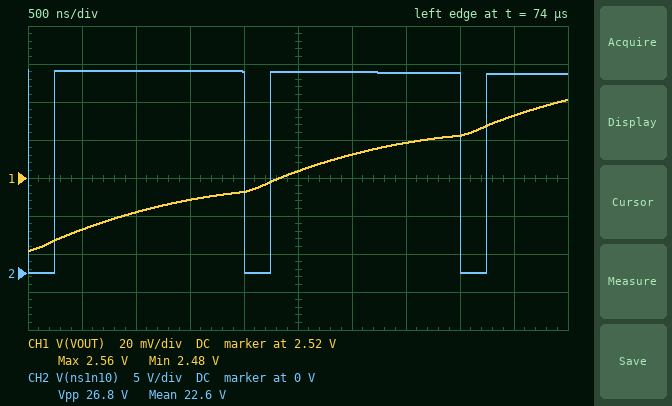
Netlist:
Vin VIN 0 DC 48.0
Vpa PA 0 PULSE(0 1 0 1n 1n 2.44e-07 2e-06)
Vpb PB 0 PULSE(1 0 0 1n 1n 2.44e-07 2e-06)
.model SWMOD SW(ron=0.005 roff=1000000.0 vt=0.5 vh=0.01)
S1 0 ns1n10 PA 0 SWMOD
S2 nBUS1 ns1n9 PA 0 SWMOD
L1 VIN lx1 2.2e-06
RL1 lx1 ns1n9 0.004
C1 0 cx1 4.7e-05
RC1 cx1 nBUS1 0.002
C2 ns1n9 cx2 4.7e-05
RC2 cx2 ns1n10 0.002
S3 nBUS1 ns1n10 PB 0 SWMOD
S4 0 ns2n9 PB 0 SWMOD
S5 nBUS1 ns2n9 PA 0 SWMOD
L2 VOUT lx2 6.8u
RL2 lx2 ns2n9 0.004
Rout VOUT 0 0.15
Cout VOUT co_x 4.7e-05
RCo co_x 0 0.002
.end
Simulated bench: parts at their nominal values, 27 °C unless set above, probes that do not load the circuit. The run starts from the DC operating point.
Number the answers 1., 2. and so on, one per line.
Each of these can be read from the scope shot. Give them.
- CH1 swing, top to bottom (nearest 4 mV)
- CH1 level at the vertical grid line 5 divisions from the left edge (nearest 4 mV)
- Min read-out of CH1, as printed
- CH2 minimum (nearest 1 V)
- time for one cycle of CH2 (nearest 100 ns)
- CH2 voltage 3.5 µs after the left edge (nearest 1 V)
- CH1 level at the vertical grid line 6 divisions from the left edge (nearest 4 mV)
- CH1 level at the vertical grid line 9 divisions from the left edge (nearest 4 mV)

1. 80 mV
2. 2.524 V
3. 2.48 V
4. 0 V
5. 2.0 µs
6. 26 V
7. 2.532 V
8. 2.552 V
